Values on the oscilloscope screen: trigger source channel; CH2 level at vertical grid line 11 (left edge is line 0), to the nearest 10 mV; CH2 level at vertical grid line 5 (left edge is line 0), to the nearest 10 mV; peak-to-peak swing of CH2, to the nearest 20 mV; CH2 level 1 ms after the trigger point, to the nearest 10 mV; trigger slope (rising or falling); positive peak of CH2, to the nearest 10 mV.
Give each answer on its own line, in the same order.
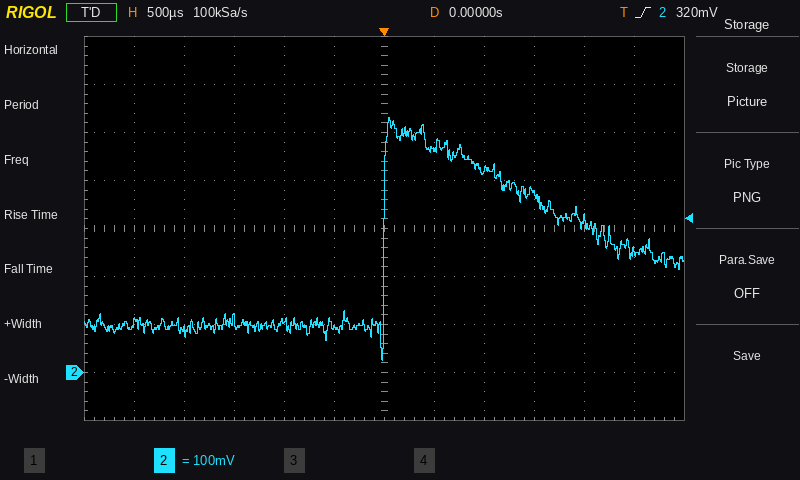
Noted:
CH2
250 mV
100 mV
500 mV
420 mV
rising
530 mV
